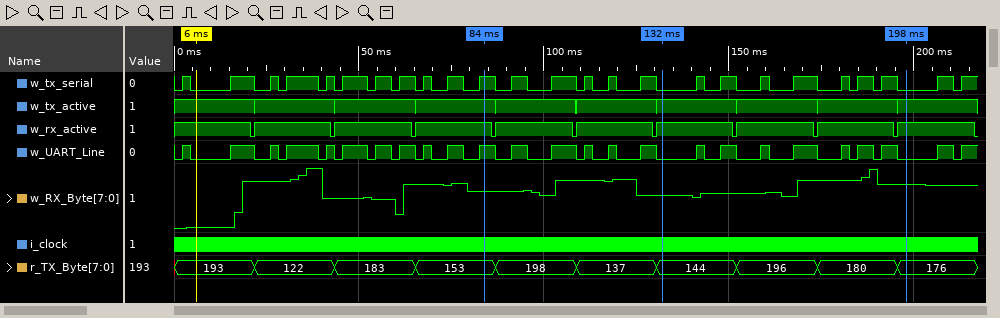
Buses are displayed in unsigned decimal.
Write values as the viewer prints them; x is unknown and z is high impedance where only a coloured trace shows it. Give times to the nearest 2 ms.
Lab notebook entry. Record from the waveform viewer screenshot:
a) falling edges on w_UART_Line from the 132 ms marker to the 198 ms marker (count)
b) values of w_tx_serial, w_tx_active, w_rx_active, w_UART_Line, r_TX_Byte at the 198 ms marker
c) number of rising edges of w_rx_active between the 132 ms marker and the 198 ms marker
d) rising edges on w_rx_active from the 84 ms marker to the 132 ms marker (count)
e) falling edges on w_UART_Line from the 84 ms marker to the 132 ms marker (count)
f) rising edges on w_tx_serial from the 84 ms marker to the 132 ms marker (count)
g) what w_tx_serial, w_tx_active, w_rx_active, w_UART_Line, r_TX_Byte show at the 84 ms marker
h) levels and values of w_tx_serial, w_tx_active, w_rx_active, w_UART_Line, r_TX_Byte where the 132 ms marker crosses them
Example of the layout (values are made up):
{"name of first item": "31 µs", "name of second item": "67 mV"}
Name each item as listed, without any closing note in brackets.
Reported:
{"falling edges on w_UART_Line from the 132 ms marker to the 198 ms marker": "7", "values of w_tx_serial, w_tx_active, w_rx_active, w_UART_Line, r_TX_Byte at the 198 ms marker": "w_tx_serial=0, w_tx_active=1, w_rx_active=1, w_UART_Line=0, r_TX_Byte=176", "number of rising edges of w_rx_active between the 132 ms marker and the 198 ms marker": "3", "rising edges on w_rx_active from the 84 ms marker to the 132 ms marker": "3", "falling edges on w_UART_Line from the 84 ms marker to the 132 ms marker": "6", "rising edges on w_tx_serial from the 84 ms marker to the 132 ms marker": "5", "what w_tx_serial, w_tx_active, w_rx_active, w_UART_Line, r_TX_Byte show at the 84 ms marker": "w_tx_serial=1, w_tx_active=1, w_rx_active=1, w_UART_Line=1, r_TX_Byte=153", "levels and values of w_tx_serial, w_tx_active, w_rx_active, w_UART_Line, r_TX_Byte where the 132 ms marker crosses them": "w_tx_serial=0, w_tx_active=1, w_rx_active=1, w_UART_Line=0, r_TX_Byte=144"}
